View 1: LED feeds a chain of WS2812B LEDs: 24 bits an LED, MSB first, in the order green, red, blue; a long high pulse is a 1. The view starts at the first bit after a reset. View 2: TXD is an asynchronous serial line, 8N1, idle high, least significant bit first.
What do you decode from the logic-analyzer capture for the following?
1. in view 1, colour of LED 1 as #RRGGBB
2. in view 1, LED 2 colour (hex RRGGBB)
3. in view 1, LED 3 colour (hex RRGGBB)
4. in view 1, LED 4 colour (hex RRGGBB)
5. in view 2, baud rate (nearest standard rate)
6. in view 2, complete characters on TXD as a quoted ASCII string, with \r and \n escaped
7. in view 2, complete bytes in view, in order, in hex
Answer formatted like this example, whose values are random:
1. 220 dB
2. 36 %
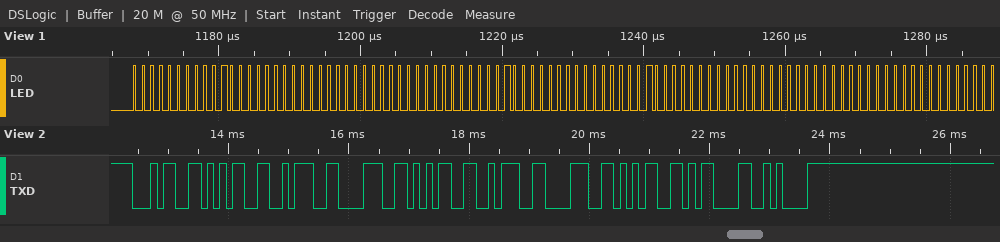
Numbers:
1. #200000
2. #000020
3. #200000
4. #000000
5. 9600 baud
6. "45:85:85\r\n"
7. 0x34 0x35 0x3A 0x38 0x35 0x3A 0x38 0x35 0x0D 0x0A
